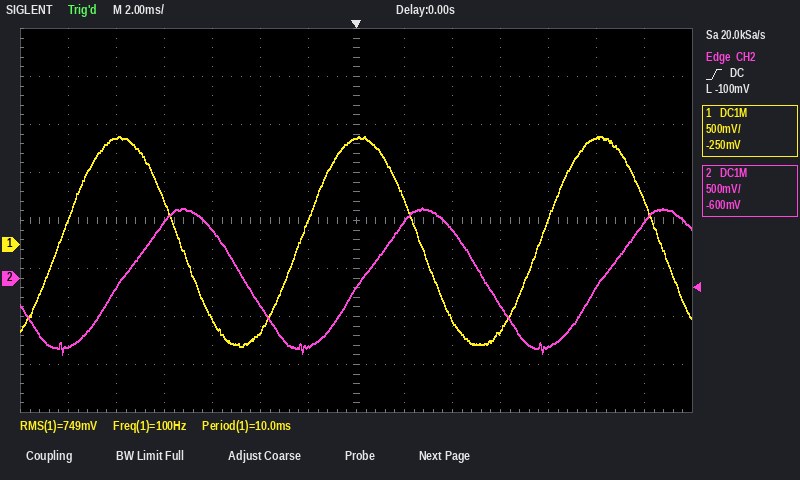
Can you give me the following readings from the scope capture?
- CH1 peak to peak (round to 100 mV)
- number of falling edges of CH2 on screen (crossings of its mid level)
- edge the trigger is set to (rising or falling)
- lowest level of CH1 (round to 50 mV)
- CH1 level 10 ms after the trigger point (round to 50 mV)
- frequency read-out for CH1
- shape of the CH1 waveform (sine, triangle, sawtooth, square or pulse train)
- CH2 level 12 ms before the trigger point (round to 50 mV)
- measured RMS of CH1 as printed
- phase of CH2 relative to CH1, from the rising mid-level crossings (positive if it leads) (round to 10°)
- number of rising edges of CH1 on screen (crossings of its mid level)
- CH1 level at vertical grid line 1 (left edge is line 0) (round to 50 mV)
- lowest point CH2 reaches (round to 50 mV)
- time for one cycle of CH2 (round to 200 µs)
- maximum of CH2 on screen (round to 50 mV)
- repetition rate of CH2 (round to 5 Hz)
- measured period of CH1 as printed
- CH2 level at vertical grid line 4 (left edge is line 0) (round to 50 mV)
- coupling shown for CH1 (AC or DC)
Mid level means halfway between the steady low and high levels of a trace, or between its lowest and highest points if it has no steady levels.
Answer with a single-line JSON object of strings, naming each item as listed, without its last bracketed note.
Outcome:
{"CH1 peak to peak": "2.20 V", "number of falling edges of CH2 on screen": "2", "edge the trigger is set to": "rising", "lowest level of CH1": "-1.05 V", "CH1 level 10 ms after the trigger point": "1.10 V", "frequency read-out for CH1": "100 Hz", "shape of the CH1 waveform": "sine", "CH2 level 12 ms before the trigger point": "-700 mV", "measured RMS of CH1 as printed": "749 mV", "phase of CH2 relative to CH1, from the rising mid-level crossings (positive if it leads)": "-90°", "number of rising edges of CH1 on screen": "3", "CH1 level at vertical grid line 1 (left edge is line 0)": "250 mV", "lowest point CH2 reaches": "-800 mV", "time for one cycle of CH2": "10.0 ms", "maximum of CH2 on screen": "750 mV", "repetition rate of CH2": "100 Hz", "measured period of CH1 as printed": "10.0 ms", "CH2 level at vertical grid line 4 (left edge is line 0)": "500 mV", "coupling shown for CH1": "DC"}
